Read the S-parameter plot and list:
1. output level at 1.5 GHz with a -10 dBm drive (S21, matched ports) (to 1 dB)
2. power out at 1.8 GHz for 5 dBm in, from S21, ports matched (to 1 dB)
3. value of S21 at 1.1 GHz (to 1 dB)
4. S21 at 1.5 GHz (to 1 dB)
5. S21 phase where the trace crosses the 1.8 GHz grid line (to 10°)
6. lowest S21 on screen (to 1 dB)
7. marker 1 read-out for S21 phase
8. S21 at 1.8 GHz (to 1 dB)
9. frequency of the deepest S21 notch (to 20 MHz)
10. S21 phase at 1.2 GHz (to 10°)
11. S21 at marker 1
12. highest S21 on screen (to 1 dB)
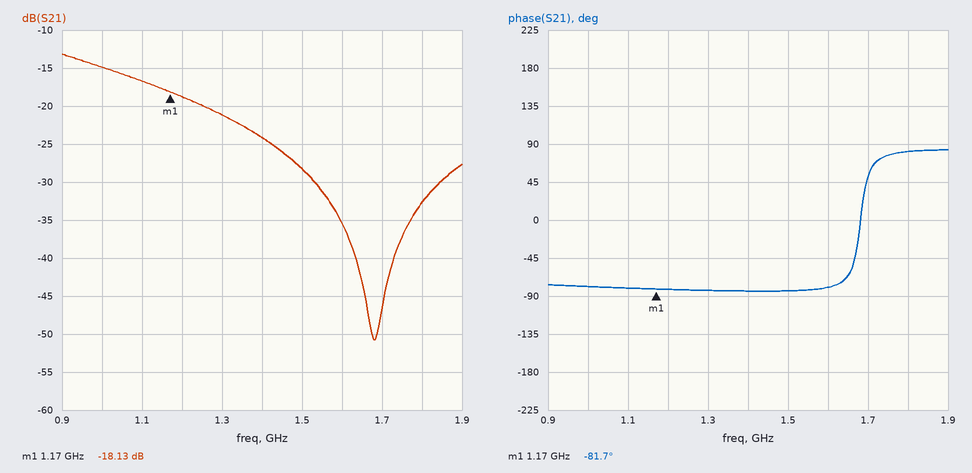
-38 dBm
-28 dBm
-17 dB
-28 dB
80°
-51 dB
-81.7°
-33 dB
1.68 GHz
-80°
-18.13 dB
-13 dB
